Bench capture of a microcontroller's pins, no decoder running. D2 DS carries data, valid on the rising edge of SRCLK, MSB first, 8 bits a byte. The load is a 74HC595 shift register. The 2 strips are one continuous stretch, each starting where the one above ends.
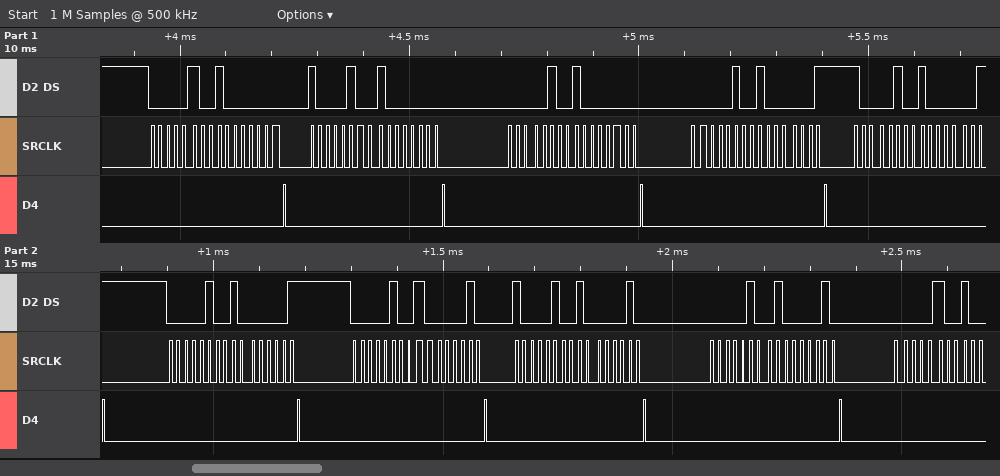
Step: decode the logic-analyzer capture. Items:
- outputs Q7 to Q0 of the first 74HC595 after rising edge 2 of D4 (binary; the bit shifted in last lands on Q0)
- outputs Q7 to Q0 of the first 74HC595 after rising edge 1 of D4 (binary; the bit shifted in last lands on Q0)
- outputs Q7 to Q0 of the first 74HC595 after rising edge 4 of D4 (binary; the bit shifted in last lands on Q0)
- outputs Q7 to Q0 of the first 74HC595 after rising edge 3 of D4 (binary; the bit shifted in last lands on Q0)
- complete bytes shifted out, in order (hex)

10000000
10000000
10000001
10000000
04 80 84 80 04 80 04 81 84 81 04 81 04 82 84 82 04 82 04
